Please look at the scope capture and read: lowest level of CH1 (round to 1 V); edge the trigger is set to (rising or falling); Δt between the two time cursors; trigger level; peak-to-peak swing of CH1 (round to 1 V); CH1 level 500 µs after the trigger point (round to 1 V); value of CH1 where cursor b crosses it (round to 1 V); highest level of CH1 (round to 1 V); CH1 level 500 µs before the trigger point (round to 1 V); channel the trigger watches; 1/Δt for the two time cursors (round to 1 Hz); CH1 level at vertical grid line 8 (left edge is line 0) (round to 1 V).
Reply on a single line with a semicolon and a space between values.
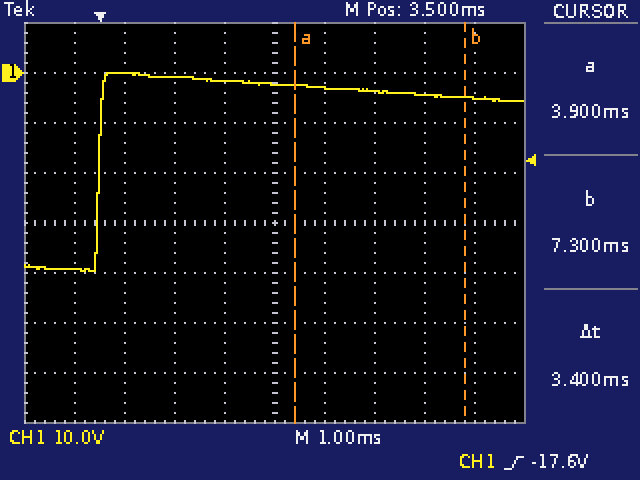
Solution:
-40 V; rising; 3.4 ms; -17.6 V; 40 V; 0 V; -5 V; 0 V; -39 V; CH1; 294 Hz; -4 V
